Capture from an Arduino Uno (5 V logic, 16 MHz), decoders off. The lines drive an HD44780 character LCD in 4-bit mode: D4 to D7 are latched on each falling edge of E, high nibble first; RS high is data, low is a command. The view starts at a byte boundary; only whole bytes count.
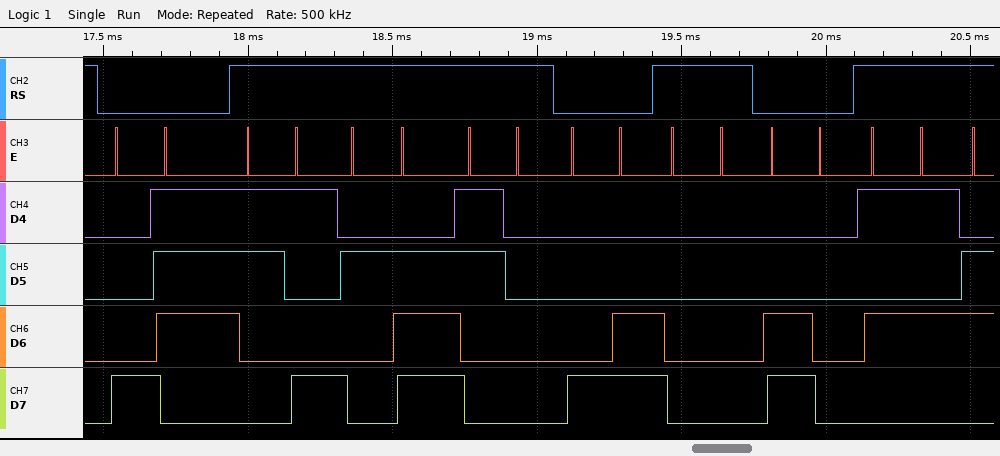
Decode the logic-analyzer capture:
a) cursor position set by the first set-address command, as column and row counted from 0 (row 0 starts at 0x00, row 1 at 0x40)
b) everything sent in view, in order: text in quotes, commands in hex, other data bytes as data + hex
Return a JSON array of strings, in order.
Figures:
["column 7, row 0", "0x87 \"9.0\" 0x8C data 00 0xC0 \"U\""]
